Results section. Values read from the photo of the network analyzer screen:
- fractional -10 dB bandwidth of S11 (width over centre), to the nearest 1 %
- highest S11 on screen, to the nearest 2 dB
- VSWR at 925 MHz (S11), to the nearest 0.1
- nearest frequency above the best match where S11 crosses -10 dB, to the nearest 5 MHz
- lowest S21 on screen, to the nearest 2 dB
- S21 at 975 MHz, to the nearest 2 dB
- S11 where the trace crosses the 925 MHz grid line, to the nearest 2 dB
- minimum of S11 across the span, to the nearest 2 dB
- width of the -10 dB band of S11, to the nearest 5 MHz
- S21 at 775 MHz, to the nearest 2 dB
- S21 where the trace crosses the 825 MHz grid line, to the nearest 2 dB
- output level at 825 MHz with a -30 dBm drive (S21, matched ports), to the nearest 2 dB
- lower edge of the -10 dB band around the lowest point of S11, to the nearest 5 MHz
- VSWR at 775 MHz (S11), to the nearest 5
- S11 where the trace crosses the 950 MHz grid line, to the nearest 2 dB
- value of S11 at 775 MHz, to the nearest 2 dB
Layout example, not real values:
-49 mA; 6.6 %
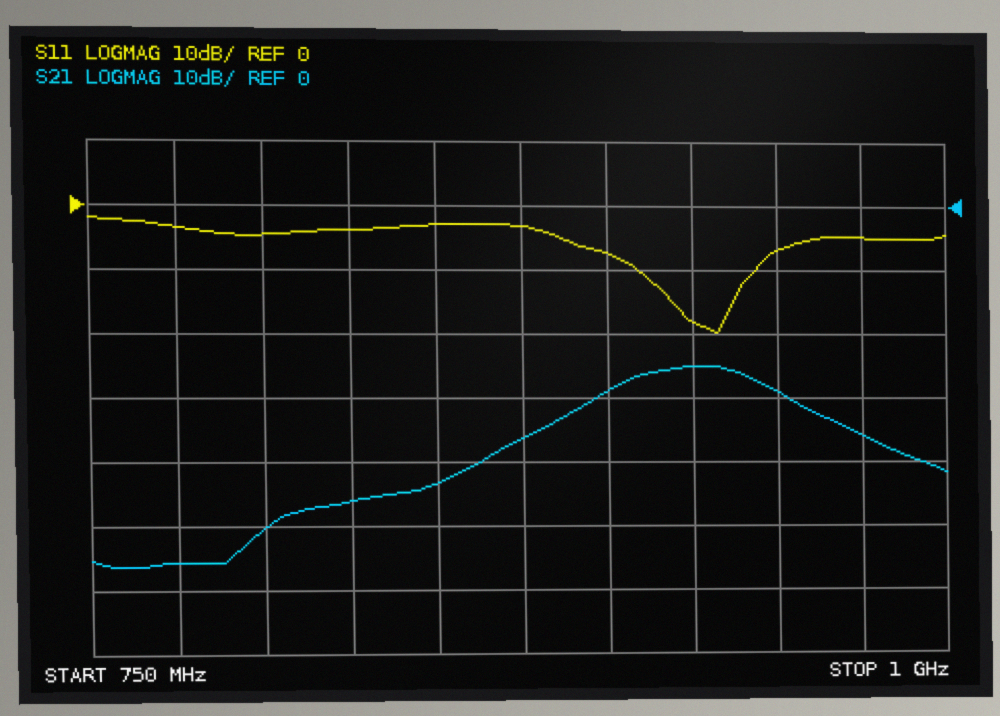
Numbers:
4 %; -2 dB; 1.3; 945 MHz; -56 dB; -36 dB; -18 dB; -20 dB; 35 MHz; -56 dB; -46 dB; -76 dBm; 910 MHz; 5; -6 dB; -4 dB
